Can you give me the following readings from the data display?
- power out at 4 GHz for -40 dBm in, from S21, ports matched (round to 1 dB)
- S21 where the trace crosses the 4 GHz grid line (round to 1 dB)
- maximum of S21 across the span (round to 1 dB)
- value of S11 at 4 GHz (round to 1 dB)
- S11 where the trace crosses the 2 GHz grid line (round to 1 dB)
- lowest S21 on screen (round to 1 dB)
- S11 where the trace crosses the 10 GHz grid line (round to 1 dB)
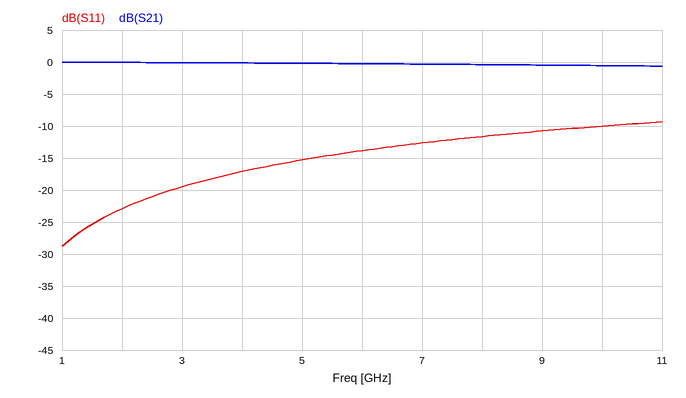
-40 dBm
0 dB
0 dB
-17 dB
-23 dB
-1 dB
-10 dB
